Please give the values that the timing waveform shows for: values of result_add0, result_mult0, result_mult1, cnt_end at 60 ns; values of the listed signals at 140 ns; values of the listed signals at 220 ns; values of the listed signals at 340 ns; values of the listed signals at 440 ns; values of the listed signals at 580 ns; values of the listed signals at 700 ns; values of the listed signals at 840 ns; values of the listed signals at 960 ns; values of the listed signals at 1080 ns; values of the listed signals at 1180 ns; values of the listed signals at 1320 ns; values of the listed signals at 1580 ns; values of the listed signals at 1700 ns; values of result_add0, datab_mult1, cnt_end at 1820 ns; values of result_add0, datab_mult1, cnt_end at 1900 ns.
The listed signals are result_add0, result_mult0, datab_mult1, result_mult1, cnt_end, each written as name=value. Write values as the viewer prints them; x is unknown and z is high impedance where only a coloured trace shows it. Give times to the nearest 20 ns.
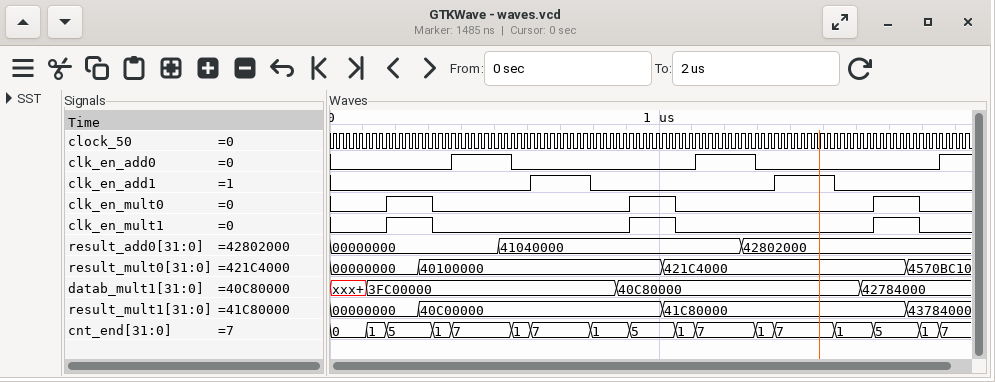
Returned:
result_add0=00000000, result_mult0=00000000, result_mult1=00000000, cnt_end=0
result_add0=00000000, result_mult0=00000000, datab_mult1=3FC00000, result_mult1=00000000, cnt_end=1
result_add0=00000000, result_mult0=00000000, datab_mult1=3FC00000, result_mult1=00000000, cnt_end=5
result_add0=00000000, result_mult0=40100000, datab_mult1=3FC00000, result_mult1=40C00000, cnt_end=1
result_add0=00000000, result_mult0=40100000, datab_mult1=3FC00000, result_mult1=40C00000, cnt_end=7
result_add0=41040000, result_mult0=40100000, datab_mult1=3FC00000, result_mult1=40C00000, cnt_end=1
result_add0=41040000, result_mult0=40100000, datab_mult1=3FC00000, result_mult1=40C00000, cnt_end=7
result_add0=41040000, result_mult0=40100000, datab_mult1=3FC00000, result_mult1=40C00000, cnt_end=1
result_add0=41040000, result_mult0=40100000, datab_mult1=40C80000, result_mult1=40C00000, cnt_end=5
result_add0=41040000, result_mult0=421C4000, datab_mult1=40C80000, result_mult1=41C80000, cnt_end=1
result_add0=41040000, result_mult0=421C4000, datab_mult1=40C80000, result_mult1=41C80000, cnt_end=7
result_add0=42802000, result_mult0=421C4000, datab_mult1=40C80000, result_mult1=41C80000, cnt_end=1
result_add0=42802000, result_mult0=421C4000, datab_mult1=40C80000, result_mult1=41C80000, cnt_end=1
result_add0=42802000, result_mult0=421C4000, datab_mult1=42784000, result_mult1=41C80000, cnt_end=5
result_add0=42802000, datab_mult1=42784000, cnt_end=1
result_add0=42802000, datab_mult1=42784000, cnt_end=7
